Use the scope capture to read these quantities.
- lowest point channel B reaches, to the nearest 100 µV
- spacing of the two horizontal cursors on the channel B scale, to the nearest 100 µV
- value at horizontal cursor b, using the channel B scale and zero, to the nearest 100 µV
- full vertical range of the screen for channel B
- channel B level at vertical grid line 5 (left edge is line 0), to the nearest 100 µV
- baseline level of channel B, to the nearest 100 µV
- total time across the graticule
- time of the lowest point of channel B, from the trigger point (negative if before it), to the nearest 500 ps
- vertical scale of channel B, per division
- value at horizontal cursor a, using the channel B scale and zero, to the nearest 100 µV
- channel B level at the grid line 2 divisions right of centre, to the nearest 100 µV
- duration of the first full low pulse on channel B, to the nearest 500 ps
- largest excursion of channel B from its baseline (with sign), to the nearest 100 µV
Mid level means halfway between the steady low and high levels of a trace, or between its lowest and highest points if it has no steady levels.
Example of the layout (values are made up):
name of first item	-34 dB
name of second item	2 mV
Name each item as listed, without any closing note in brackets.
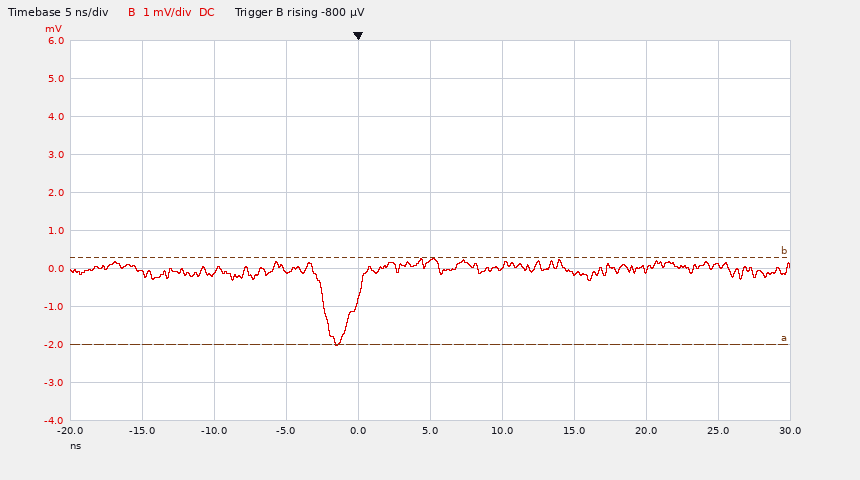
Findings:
lowest point channel B reaches, to the nearest 100 µV	-2.0 mV
spacing of the two horizontal cursors on the channel B scale, to the nearest 100 µV	2.3 mV
value at horizontal cursor b, using the channel B scale and zero, to the nearest 100 µV	300 µV
full vertical range of the screen for channel B	10 mV
channel B level at vertical grid line 5 (left edge is line 0), to the nearest 100 µV	200 µV
baseline level of channel B, to the nearest 100 µV	0.0 mV
total time across the graticule	50 ns
time of the lowest point of channel B, from the trigger point (negative if before it), to the nearest 500 ps	-1.5 ns
vertical scale of channel B, per division	1 mV
value at horizontal cursor a, using the channel B scale and zero, to the nearest 100 µV	-2.0 mV
channel B level at the grid line 2 divisions right of centre, to the nearest 100 µV	-100 µV
duration of the first full low pulse on channel B, to the nearest 500 ps	2.5 ns
largest excursion of channel B from its baseline (with sign), to the nearest 100 µV	-2.0 mV
